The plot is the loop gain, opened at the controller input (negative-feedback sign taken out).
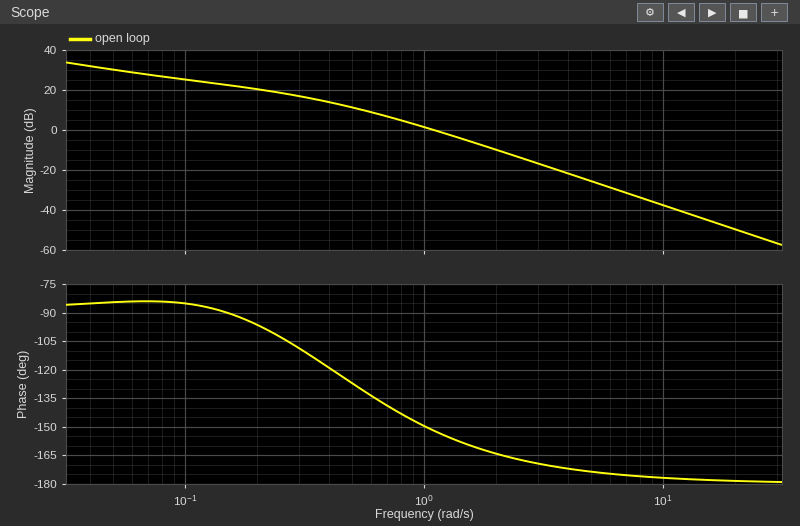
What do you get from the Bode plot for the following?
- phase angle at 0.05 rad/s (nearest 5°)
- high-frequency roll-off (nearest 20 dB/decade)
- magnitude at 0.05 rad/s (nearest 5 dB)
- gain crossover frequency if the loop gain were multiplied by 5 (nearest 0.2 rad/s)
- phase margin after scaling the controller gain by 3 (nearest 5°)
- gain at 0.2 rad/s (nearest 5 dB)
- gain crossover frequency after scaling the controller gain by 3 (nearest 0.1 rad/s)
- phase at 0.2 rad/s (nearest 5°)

-85°
-40 dB/decade
30 dB
2.6 rad/s
15°
20 dB
2.0 rad/s
-95°
